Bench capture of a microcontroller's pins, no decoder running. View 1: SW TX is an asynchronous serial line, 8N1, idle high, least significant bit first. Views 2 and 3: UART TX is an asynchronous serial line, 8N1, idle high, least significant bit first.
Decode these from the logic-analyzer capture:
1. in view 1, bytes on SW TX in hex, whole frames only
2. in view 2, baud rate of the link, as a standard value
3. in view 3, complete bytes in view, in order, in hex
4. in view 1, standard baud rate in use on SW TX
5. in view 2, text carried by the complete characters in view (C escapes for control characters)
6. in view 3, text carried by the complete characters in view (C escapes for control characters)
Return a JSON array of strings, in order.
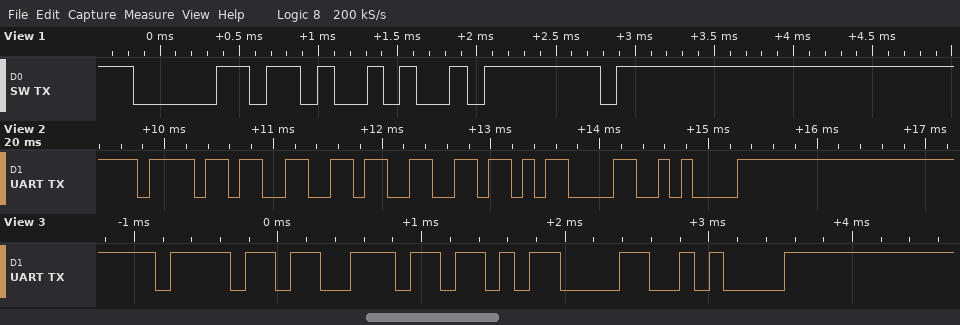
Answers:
["0xB0 0x29 0x7F", "9600 baud", "6F 6E 0D 0A", "9600 baud", "\"off\\r\\n\"", "\"on\\r\\n\""]
